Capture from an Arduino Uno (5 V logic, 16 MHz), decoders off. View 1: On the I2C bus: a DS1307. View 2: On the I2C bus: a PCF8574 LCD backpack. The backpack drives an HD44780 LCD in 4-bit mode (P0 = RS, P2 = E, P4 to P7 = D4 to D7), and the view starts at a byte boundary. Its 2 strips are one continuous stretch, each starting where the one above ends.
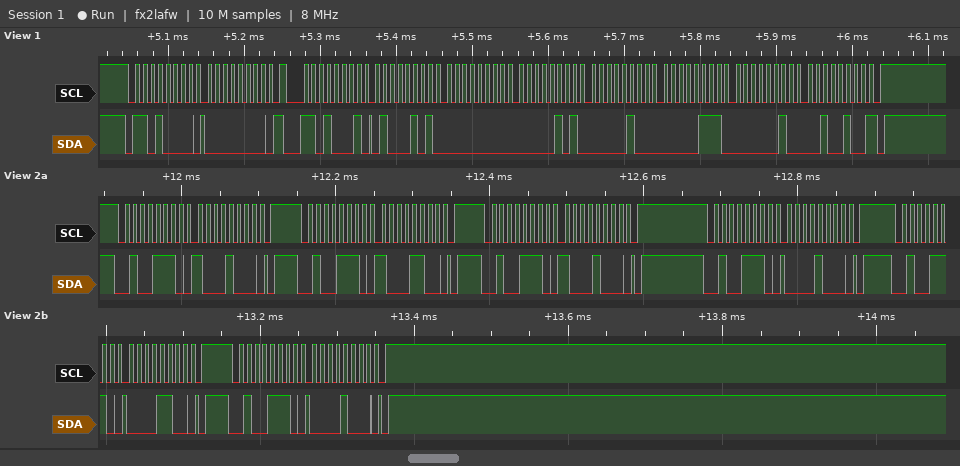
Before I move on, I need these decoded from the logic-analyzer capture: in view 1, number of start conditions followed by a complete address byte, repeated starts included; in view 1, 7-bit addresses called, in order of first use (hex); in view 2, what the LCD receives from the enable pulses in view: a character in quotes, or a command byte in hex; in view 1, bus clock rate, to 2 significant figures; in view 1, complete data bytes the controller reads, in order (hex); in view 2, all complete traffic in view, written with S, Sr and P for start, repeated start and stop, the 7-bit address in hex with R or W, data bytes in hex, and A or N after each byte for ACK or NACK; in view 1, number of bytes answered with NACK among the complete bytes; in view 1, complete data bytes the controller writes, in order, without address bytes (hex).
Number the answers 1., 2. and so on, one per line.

1. 2
2. 0x68
3. 0x80
4. 100 kHz
5. 45 00 05 04 07 02 24
6. S 27W A 88 A P S 27W A 8C A P S 27W A 88 A P S 27W A 08 A P S 27W A 0C A P S 27W A 08 A P
7. 1
8. 00
